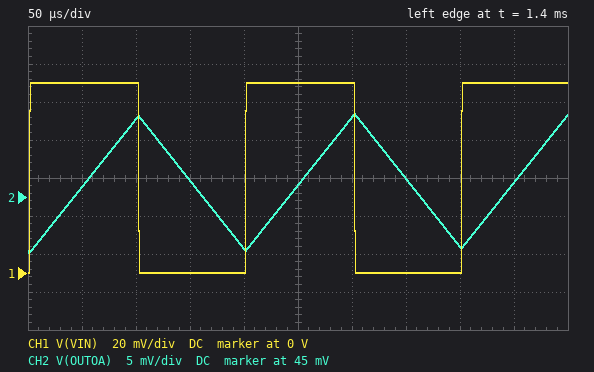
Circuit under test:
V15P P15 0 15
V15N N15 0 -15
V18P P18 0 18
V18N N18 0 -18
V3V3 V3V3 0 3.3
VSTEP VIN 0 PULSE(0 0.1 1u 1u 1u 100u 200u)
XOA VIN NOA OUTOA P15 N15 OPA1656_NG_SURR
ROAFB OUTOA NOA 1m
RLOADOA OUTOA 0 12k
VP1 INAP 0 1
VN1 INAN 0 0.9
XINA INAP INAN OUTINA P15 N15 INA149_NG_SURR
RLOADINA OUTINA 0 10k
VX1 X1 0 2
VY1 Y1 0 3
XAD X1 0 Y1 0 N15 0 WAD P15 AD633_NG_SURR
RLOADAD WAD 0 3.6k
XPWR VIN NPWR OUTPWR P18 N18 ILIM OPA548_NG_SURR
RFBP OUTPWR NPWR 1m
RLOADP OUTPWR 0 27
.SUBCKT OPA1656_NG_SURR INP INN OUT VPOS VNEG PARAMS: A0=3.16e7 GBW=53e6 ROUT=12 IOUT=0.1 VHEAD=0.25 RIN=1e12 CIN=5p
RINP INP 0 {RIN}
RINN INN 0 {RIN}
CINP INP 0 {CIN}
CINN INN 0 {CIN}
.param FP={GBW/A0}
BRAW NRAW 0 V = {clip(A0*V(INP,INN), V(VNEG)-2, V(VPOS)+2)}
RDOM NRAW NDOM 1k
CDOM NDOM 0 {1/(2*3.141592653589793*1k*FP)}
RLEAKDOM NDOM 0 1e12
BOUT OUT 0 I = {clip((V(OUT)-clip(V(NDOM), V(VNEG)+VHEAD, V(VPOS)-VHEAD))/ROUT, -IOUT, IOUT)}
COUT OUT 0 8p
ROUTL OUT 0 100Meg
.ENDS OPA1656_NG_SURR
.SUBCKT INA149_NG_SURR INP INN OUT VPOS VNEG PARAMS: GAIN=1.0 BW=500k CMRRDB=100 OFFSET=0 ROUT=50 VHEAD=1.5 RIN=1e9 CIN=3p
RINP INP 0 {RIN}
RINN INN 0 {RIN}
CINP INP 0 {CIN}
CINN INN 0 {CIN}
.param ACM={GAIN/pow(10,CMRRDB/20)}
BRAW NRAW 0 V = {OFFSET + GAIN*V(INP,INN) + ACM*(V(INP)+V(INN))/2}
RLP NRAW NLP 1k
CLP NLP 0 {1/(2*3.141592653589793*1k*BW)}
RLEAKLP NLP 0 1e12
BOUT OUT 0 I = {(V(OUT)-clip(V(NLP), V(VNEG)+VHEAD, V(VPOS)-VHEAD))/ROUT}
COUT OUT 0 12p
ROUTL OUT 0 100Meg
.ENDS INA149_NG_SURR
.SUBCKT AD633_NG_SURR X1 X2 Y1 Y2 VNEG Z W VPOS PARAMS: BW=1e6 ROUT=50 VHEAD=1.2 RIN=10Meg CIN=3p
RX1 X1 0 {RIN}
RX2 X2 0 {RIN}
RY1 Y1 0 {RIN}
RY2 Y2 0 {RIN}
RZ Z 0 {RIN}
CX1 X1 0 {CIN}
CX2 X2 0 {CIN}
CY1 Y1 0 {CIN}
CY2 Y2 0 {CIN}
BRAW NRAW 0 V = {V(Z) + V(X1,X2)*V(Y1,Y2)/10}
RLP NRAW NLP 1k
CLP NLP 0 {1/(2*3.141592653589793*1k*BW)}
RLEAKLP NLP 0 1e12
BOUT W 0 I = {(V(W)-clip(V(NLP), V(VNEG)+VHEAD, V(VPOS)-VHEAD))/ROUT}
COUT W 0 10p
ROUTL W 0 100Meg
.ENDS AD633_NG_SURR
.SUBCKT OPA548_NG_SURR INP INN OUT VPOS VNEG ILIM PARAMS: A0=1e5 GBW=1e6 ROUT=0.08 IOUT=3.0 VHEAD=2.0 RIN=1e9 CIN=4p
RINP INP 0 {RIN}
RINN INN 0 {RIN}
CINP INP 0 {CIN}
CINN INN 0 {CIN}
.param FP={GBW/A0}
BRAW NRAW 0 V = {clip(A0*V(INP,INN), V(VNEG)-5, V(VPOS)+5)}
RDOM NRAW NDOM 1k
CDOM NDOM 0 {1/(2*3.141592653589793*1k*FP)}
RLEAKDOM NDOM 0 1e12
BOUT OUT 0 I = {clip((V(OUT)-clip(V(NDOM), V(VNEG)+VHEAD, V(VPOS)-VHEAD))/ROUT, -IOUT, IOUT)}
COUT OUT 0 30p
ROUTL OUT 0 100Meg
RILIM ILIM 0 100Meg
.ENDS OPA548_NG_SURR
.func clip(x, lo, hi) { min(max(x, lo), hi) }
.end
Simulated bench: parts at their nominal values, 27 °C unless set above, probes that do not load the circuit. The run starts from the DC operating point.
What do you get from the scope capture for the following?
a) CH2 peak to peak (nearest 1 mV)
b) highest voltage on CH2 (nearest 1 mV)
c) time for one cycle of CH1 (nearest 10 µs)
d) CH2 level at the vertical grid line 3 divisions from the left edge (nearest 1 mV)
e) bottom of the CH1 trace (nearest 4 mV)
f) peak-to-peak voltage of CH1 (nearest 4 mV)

18 mV
56 mV
200 µs
47 mV
0 V
100 mV
